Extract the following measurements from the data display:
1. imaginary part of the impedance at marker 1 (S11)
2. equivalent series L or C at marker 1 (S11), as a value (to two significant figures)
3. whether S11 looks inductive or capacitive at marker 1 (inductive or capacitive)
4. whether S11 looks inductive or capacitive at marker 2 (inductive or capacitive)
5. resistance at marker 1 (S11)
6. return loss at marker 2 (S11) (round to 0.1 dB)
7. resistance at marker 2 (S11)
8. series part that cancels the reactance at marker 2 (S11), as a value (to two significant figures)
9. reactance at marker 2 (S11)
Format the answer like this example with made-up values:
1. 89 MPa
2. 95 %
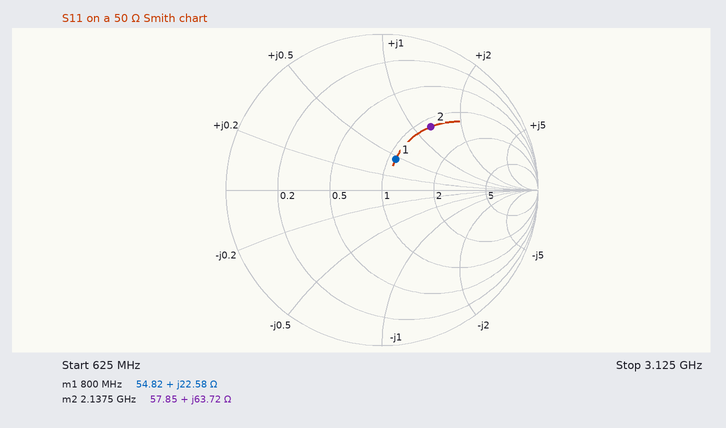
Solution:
1. +22.58 Ω
2. 4.5 nH
3. inductive
4. inductive
5. 54.82 Ω
6. 5.8 dB
7. 57.85 Ω
8. 1.2 pF
9. +63.72 Ω
